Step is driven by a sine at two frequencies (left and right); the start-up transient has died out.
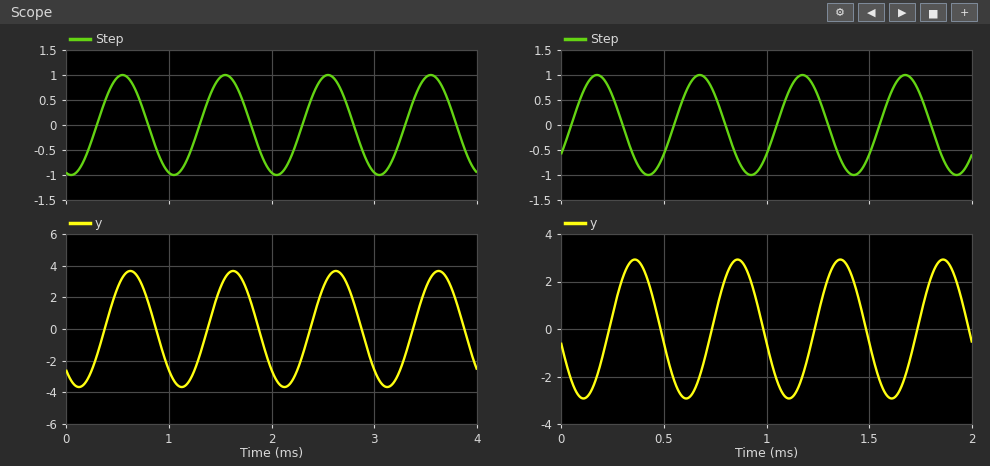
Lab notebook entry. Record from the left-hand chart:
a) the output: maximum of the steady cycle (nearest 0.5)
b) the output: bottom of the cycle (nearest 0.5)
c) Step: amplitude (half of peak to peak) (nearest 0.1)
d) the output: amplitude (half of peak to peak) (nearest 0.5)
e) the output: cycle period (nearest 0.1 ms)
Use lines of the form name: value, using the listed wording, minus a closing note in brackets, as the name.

the output: maximum of the steady cycle: 3.5
the output: bottom of the cycle: -3.5
Step: amplitude (half of peak to peak): 1.0
the output: amplitude (half of peak to peak): 3.5
the output: cycle period: 1.0 ms
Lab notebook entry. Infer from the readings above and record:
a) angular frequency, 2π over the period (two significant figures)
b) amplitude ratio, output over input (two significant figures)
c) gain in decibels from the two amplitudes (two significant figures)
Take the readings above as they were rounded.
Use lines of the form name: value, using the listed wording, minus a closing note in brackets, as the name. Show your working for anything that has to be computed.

angular frequency, 2π over the period: 2π / 1 = 6.3 rad/ms
amplitude ratio, output over input: 3.5 / 1 = 3.5
gain in decibels from the two amplitudes: 20 log10(3.5 / 1) = 11 dB
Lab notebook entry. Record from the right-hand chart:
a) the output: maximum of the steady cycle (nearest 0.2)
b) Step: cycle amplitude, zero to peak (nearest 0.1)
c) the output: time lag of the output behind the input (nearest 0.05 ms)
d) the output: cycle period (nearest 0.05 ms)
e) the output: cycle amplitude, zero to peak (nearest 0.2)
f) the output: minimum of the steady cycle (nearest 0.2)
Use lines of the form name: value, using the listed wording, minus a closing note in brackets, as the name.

the output: maximum of the steady cycle: 3.0
Step: cycle amplitude, zero to peak: 1.0
the output: time lag of the output behind the input: 0.20 ms
the output: cycle period: 0.50 ms
the output: cycle amplitude, zero to peak: 3.0
the output: minimum of the steady cycle: -3.0
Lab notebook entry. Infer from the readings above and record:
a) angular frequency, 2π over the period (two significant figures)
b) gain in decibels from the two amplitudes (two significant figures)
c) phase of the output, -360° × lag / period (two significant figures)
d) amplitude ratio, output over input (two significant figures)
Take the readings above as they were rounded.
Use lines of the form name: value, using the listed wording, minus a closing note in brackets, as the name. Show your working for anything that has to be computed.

angular frequency, 2π over the period: 2π / 0.5 = 13 rad/ms
gain in decibels from the two amplitudes: 20 log10(3 / 1) = 9.5 dB
phase of the output, -360° × lag / period: -360 × 0.2 / 0.5 = -140°
amplitude ratio, output over input: 3 / 1 = 3.0
